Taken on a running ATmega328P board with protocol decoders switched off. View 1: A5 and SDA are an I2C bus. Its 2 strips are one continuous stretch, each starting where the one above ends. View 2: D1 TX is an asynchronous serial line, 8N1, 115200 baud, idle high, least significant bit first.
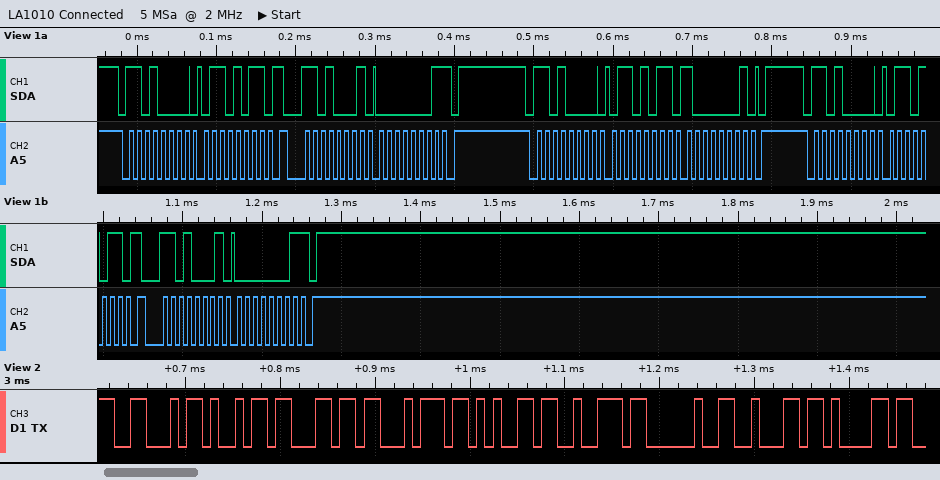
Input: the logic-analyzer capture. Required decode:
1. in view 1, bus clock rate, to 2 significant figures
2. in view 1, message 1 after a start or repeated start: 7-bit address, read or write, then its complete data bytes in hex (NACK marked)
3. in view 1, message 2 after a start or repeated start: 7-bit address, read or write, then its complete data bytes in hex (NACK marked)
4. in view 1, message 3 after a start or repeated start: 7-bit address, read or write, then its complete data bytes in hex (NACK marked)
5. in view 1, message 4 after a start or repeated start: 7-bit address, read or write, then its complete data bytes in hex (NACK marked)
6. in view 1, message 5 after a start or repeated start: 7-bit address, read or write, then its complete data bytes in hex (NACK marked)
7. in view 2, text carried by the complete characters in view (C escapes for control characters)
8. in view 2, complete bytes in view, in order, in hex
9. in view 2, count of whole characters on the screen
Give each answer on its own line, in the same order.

100 kHz
0x68 write: 6B
0x68 read: 01 NACK
0x68 write: 6B 81
0x68 write: 6B
0x68 read: 01 NACK
"Filter ba"
46 69 6C 74 65 72 20 62 61
9
